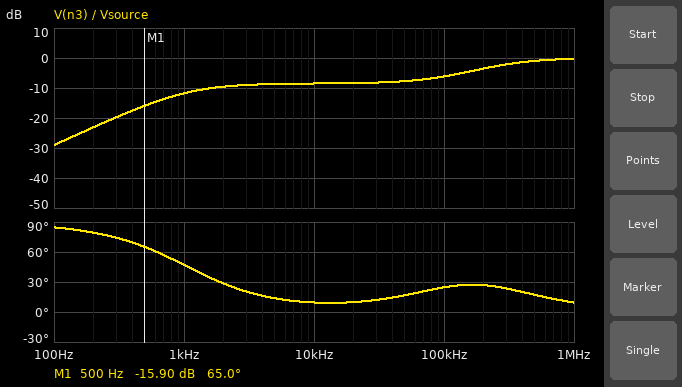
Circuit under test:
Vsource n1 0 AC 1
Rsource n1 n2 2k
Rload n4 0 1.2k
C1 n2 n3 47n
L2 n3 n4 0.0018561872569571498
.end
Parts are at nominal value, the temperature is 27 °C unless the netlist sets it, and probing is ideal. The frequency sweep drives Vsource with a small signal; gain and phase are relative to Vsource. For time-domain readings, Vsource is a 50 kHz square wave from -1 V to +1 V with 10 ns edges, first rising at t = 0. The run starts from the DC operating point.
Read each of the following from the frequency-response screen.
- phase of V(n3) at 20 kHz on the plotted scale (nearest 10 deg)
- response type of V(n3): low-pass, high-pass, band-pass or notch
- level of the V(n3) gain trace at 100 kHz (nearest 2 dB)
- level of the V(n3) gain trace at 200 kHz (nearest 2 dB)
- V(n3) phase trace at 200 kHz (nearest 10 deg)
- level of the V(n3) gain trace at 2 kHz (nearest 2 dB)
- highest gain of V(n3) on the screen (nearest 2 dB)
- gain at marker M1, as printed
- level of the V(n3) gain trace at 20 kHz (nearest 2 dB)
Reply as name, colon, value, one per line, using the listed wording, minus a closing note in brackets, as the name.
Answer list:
phase of V(n3) at 20 kHz on the plotted scale: 10 deg
response type of V(n3): low-pass, high-pass, band-pass or notch: high-pass
level of the V(n3) gain trace at 100 kHz: -6 dB
level of the V(n3) gain trace at 200 kHz: -4 dB
V(n3) phase trace at 200 kHz: 30 deg
level of the V(n3) gain trace at 2 kHz: -10 dB
highest gain of V(n3) on the screen: 0 dB
gain at marker M1, as printed: -15.90 dB
level of the V(n3) gain trace at 20 kHz: -8 dB
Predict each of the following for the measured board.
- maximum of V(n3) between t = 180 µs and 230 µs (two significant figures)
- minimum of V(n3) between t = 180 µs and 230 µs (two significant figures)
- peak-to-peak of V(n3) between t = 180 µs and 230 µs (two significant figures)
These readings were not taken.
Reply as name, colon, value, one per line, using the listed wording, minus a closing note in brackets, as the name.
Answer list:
maximum of V(n3) between t = 180 µs and 230 µs: 1.7 V
minimum of V(n3) between t = 180 µs and 230 µs: -1.5 V
peak-to-peak of V(n3) between t = 180 µs and 230 µs: 3.3 V
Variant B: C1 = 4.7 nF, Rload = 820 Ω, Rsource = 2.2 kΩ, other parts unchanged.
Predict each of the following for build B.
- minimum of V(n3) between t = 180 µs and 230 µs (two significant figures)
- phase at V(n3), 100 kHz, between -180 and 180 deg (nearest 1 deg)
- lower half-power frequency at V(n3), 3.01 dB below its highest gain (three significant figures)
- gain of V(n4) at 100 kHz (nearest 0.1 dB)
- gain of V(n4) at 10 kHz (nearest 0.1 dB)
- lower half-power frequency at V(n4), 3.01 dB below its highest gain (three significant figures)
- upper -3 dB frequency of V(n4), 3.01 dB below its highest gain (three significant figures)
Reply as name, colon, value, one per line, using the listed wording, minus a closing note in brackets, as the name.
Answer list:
minimum of V(n3) between t = 180 µs and 230 µs: -1.8 V
phase at V(n3), 100 kHz, between -180 and 180 deg: 40 deg
lower half-power frequency at V(n3), 3.01 dB below its highest gain: 227 kHz
gain of V(n4) at 100 kHz: -11.6 dB
gain of V(n4) at 10 kHz: -14.7 dB
lower half-power frequency at V(n4), 3.01 dB below its highest gain: 10.8 kHz
upper -3 dB frequency of V(n4), 3.01 dB below its highest gain: 270 kHz
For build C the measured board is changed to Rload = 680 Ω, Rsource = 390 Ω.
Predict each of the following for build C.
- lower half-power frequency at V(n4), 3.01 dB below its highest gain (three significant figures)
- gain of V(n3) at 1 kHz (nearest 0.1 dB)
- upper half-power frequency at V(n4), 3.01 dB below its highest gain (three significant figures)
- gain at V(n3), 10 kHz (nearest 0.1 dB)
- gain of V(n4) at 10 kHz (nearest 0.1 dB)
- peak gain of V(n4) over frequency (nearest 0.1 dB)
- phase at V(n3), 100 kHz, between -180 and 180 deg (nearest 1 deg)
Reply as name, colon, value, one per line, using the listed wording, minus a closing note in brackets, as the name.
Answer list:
lower half-power frequency at V(n4), 3.01 dB below its highest gain: 3.06 kHz
gain of V(n3) at 1 kHz: -14.3 dB
upper half-power frequency at V(n4), 3.01 dB below its highest gain: 94.8 kHz
gain at V(n3), 10 kHz: -4.0 dB
gain of V(n4) at 10 kHz: -4.1 dB
peak gain of V(n4) over frequency: -3.9 dB
phase at V(n3), 100 kHz, between -180 and 180 deg: 13 deg
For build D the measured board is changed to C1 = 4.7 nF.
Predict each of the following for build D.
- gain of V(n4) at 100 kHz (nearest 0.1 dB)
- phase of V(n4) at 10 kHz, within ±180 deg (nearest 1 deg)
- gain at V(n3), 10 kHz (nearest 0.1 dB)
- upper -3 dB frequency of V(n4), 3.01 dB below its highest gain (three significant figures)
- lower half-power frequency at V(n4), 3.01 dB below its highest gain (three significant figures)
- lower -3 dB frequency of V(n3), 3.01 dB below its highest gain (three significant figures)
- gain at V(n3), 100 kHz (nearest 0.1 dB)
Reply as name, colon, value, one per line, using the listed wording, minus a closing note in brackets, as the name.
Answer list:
gain of V(n4) at 100 kHz: -8.8 dB
phase of V(n4) at 10 kHz, within ±180 deg: 46 deg
gain at V(n3), 10 kHz: -11.6 dB
upper -3 dB frequency of V(n4), 3.01 dB below its highest gain: 285 kHz
lower half-power frequency at V(n4), 3.01 dB below its highest gain: 10.2 kHz
lower -3 dB frequency of V(n3), 3.01 dB below its highest gain: 220 kHz
gain at V(n3), 100 kHz: -5.9 dB
